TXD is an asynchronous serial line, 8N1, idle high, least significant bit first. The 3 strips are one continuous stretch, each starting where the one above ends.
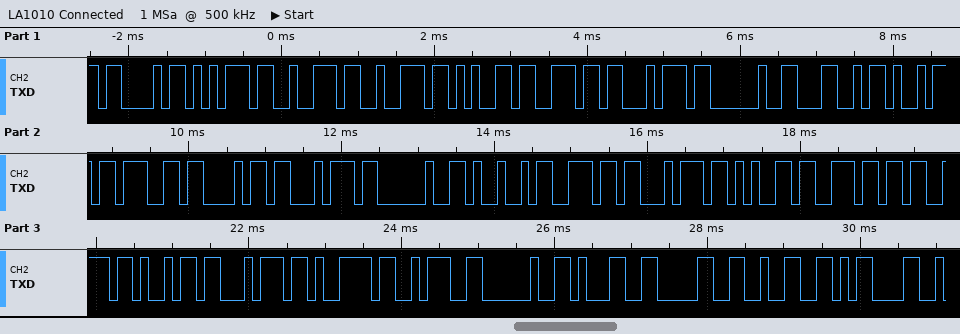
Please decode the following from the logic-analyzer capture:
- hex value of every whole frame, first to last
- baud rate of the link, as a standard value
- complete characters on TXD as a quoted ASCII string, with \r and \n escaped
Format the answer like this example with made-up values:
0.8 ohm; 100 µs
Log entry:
0x43 0x75 0x72 0x72 0x65 0x6E 0x74 0x20 0x4C 0x69 0x67 0x68 0x74 0x20 0x49 0x6E 0x74 0x65 0x6E 0x73 0x69 0x74 0x79 0x3A 0x20 0x31 0x30 0x32 0x0D; 9600 baud; "Current Light Intensity: 102\r"
